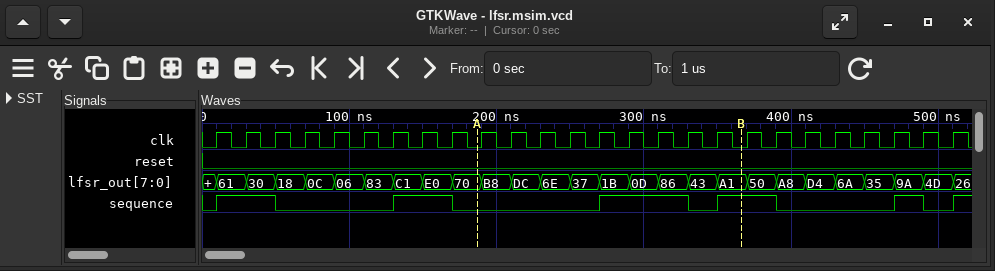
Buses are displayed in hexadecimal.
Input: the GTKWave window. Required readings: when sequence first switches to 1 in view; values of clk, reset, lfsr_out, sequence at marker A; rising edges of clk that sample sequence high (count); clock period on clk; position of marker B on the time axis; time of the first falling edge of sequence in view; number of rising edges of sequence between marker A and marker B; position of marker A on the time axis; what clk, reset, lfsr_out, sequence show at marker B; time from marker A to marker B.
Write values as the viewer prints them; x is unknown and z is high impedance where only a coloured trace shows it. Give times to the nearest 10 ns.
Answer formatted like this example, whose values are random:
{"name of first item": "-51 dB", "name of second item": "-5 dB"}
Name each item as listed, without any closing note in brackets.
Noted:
{"when sequence first switches to 1 in view": "10 ns", "values of clk, reset, lfsr_out, sequence at marker A": "clk=0, reset=0, lfsr_out=70, sequence=0", "rising edges of clk that sample sequence high": "10", "clock period on clk": "20 ns", "position of marker B on the time axis": "370 ns", "time of the first falling edge of sequence in view": "50 ns", "number of rising edges of sequence between marker A and marker B": "2", "position of marker A on the time axis": "190 ns", "what clk, reset, lfsr_out, sequence show at marker B": "clk=0, reset=0, lfsr_out=A1, sequence=1", "time from marker A to marker B": "180 ns"}
